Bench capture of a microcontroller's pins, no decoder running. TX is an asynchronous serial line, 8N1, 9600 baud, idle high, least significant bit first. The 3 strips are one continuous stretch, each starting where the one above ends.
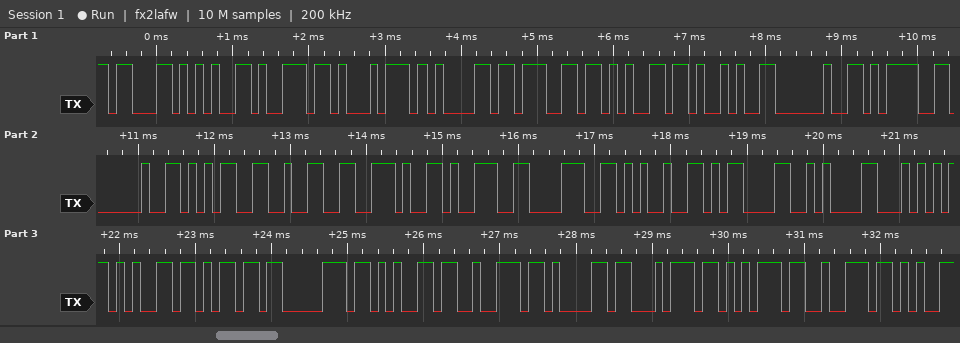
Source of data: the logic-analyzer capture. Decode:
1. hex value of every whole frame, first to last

63 65 6E 74 61 67 65 29 20 3D 20 35 32 2E 39 38 25 0D 0A 54 65 6D 70 65 72 61 74 75 72
